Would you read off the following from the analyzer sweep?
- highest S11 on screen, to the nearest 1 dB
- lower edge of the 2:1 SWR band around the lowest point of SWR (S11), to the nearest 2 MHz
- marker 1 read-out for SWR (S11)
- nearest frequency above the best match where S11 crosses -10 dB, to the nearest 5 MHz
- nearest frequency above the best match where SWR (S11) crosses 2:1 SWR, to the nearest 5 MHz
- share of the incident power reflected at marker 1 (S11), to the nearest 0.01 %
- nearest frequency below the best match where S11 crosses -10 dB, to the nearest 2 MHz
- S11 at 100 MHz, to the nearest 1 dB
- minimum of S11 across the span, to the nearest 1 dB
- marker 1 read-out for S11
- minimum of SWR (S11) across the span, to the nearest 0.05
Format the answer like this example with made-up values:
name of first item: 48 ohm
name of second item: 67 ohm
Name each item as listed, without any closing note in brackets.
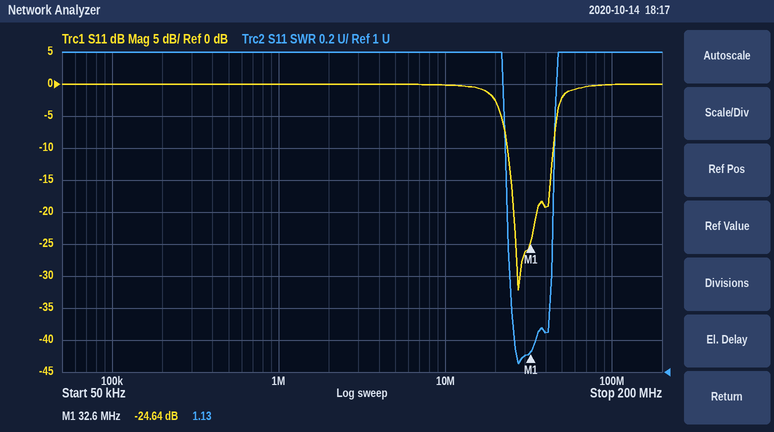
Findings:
highest S11 on screen, to the nearest 1 dB: 0 dB
lower edge of the 2:1 SWR band around the lowest point of SWR (S11), to the nearest 2 MHz: 24 MHz
marker 1 read-out for SWR: 1.13
nearest frequency above the best match where S11 crosses -10 dB, to the nearest 5 MHz: 45 MHz
nearest frequency above the best match where SWR (S11) crosses 2:1 SWR, to the nearest 5 MHz: 45 MHz
share of the incident power reflected at marker 1 (S11), to the nearest 0.01 %: 0.34 %
nearest frequency below the best match where S11 crosses -10 dB, to the nearest 2 MHz: 24 MHz
S11 at 100 MHz, to the nearest 1 dB: 0 dB
minimum of S11 across the span, to the nearest 1 dB: -32 dB
marker 1 read-out for S11: -24.64 dB
minimum of SWR (S11) across the span, to the nearest 0.05: 1.05
